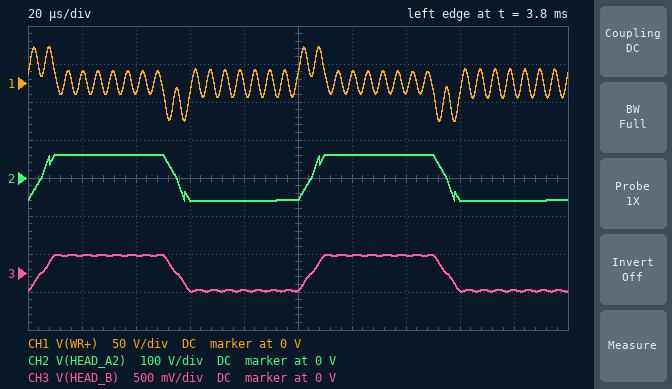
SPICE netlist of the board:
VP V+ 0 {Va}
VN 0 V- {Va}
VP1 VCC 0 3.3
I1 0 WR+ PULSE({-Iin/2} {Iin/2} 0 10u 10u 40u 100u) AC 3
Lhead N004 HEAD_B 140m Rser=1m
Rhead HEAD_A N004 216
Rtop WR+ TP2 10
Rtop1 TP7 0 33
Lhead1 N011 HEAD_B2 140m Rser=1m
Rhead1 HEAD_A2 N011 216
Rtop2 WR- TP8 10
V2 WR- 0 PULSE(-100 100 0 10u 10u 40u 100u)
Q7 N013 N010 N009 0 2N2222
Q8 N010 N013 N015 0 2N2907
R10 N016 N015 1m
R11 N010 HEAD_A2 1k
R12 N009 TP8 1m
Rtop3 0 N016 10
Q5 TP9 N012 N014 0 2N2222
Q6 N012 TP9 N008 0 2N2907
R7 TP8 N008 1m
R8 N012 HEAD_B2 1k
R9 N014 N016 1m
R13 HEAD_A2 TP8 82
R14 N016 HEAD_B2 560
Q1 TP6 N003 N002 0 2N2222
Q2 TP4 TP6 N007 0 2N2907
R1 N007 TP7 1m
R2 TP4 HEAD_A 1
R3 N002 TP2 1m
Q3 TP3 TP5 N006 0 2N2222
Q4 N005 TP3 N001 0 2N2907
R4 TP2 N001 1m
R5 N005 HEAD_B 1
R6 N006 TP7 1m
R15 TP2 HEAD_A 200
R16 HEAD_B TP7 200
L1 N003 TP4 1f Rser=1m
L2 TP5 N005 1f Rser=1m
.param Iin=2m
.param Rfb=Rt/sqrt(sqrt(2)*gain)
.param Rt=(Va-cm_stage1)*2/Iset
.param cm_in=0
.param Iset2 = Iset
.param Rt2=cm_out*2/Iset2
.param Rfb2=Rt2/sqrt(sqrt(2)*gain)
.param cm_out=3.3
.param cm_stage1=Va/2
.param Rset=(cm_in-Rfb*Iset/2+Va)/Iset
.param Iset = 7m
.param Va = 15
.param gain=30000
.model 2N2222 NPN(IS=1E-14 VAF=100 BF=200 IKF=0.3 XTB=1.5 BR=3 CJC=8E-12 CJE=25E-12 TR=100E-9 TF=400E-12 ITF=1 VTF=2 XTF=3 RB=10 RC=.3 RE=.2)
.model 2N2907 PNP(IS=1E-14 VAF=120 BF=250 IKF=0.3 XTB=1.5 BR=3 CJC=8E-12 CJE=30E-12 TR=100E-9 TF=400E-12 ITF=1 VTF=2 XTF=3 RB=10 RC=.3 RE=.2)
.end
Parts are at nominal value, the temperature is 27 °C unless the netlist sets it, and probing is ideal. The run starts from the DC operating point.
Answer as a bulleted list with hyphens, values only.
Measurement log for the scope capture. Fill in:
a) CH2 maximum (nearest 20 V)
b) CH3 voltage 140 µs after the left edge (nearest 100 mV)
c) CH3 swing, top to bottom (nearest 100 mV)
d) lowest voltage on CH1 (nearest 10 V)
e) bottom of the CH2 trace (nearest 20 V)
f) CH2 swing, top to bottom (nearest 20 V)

- 60 V
- 200 mV
- 500 mV
- -50 V
- -60 V
- 120 V
